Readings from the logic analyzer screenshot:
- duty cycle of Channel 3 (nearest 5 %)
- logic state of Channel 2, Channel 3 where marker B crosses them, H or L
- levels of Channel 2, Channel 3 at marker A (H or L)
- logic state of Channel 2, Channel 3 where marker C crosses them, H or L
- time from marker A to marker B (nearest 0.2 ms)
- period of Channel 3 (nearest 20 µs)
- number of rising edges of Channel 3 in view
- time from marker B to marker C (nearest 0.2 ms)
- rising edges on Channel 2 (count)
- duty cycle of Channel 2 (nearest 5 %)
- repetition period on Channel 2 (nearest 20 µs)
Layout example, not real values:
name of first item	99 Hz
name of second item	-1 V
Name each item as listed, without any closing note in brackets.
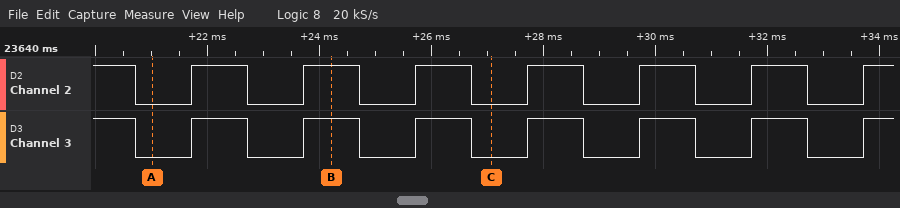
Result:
duty cycle of Channel 3	50 %
logic state of Channel 2, Channel 3 where marker B crosses them, H or L	Channel 2=H, Channel 3=H
levels of Channel 2, Channel 3 at marker A	Channel 2=L, Channel 3=L
logic state of Channel 2, Channel 3 where marker C crosses them, H or L	Channel 2=L, Channel 3=L
time from marker A to marker B	3.2 ms
period of Channel 3	2000 µs
number of rising edges of Channel 3 in view	7
time from marker B to marker C	2.8 ms
rising edges on Channel 2	7
duty cycle of Channel 2	50 %
repetition period on Channel 2	2000 µs
